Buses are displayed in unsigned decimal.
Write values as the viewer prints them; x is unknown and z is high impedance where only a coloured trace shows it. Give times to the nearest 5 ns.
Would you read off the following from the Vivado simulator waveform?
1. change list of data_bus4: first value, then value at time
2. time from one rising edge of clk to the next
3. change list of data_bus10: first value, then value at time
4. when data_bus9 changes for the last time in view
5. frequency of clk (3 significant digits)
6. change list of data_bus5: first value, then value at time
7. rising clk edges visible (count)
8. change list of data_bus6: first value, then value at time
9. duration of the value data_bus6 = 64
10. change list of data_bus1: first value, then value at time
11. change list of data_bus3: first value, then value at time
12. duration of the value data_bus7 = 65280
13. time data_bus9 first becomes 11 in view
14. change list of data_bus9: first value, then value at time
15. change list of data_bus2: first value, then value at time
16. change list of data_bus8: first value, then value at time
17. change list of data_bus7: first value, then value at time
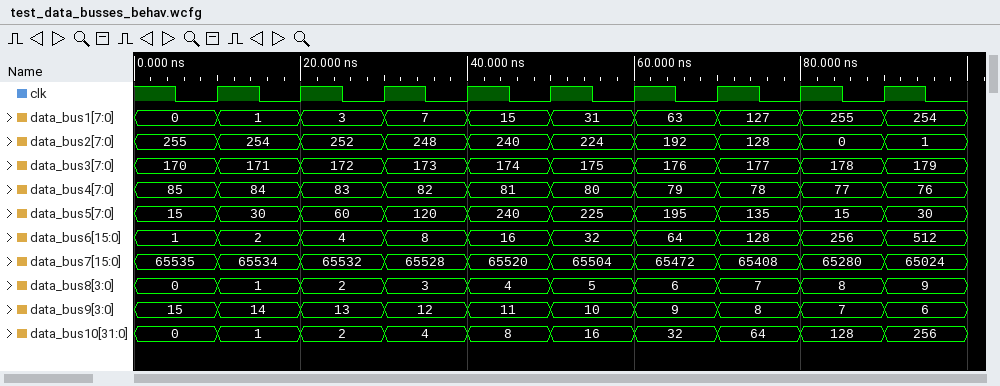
85, 84 at 10 ns, 83 at 20 ns, 82 at 30 ns, 81 at 40 ns, 80 at 50 ns, 79 at 60 ns, 78 at 70 ns, 77 at 80 ns, 76 at 90 ns
10 ns
0, 1 at 10 ns, 2 at 20 ns, 4 at 30 ns, 8 at 40 ns, 16 at 50 ns, 32 at 60 ns, 64 at 70 ns, 128 at 80 ns, 256 at 90 ns
90 ns
100 MHz
15, 30 at 10 ns, 60 at 20 ns, 120 at 30 ns, 240 at 40 ns, 225 at 50 ns, 195 at 60 ns, 135 at 70 ns, 15 at 80 ns, 30 at 90 ns
9
1, 2 at 10 ns, 4 at 20 ns, 8 at 30 ns, 16 at 40 ns, 32 at 50 ns, 64 at 60 ns, 128 at 70 ns, 256 at 80 ns, 512 at 90 ns
10 ns
0, 1 at 10 ns, 3 at 20 ns, 7 at 30 ns, 15 at 40 ns, 31 at 50 ns, 63 at 60 ns, 127 at 70 ns, 255 at 80 ns, 254 at 90 ns
170, 171 at 10 ns, 172 at 20 ns, 173 at 30 ns, 174 at 40 ns, 175 at 50 ns, 176 at 60 ns, 177 at 70 ns, 178 at 80 ns, 179 at 90 ns
10 ns
40 ns
15, 14 at 10 ns, 13 at 20 ns, 12 at 30 ns, 11 at 40 ns, 10 at 50 ns, 9 at 60 ns, 8 at 70 ns, 7 at 80 ns, 6 at 90 ns
255, 254 at 10 ns, 252 at 20 ns, 248 at 30 ns, 240 at 40 ns, 224 at 50 ns, 192 at 60 ns, 128 at 70 ns, 0 at 80 ns, 1 at 90 ns
0, 1 at 10 ns, 2 at 20 ns, 3 at 30 ns, 4 at 40 ns, 5 at 50 ns, 6 at 60 ns, 7 at 70 ns, 8 at 80 ns, 9 at 90 ns
65535, 65534 at 10 ns, 65532 at 20 ns, 65528 at 30 ns, 65520 at 40 ns, 65504 at 50 ns, 65472 at 60 ns, 65408 at 70 ns, 65280 at 80 ns, 65024 at 90 ns
